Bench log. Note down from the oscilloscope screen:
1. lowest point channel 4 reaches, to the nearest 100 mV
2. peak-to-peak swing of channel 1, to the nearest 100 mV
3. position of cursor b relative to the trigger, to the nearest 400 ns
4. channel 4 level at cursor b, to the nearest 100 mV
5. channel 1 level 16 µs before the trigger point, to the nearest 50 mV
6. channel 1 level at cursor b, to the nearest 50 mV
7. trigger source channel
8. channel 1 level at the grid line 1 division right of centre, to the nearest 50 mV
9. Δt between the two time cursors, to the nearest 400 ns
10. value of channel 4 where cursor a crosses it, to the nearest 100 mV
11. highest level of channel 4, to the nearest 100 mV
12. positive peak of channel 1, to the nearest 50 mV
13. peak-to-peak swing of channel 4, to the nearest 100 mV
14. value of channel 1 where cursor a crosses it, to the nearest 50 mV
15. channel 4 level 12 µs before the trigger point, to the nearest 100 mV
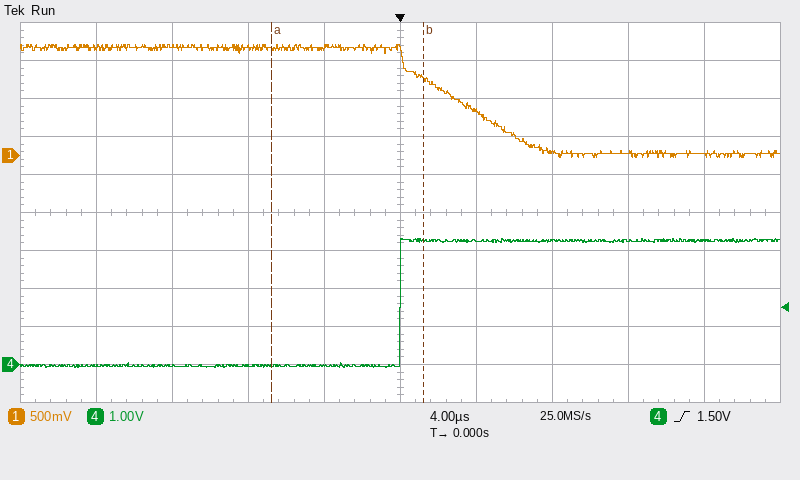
-100 mV
1.50 V
+1.2 µs
3.3 V
1.40 V
1.00 V
channel 4
600 mV
8.0 µs
0.0 V
3.3 V
1.45 V
3.4 V
1.40 V
0.0 V
